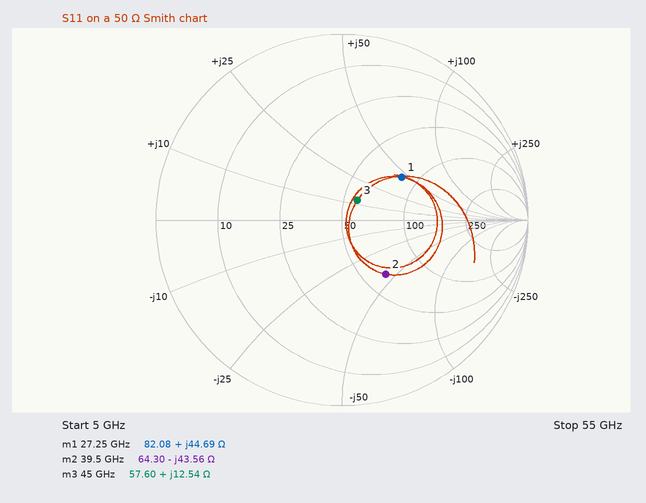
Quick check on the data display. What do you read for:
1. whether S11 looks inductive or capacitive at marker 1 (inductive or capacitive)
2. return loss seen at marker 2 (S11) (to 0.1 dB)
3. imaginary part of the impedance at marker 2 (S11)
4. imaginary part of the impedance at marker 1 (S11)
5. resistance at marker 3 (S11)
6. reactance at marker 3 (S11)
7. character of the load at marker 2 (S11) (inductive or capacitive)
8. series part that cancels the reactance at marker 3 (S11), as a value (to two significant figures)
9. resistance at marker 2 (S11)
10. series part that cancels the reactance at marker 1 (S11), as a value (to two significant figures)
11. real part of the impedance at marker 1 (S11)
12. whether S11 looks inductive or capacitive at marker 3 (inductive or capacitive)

inductive
8.5 dB
-43.56 Ω
+44.69 Ω
57.60 Ω
+12.54 Ω
capacitive
280 fF
64.30 Ω
130 fF
82.08 Ω
inductive
